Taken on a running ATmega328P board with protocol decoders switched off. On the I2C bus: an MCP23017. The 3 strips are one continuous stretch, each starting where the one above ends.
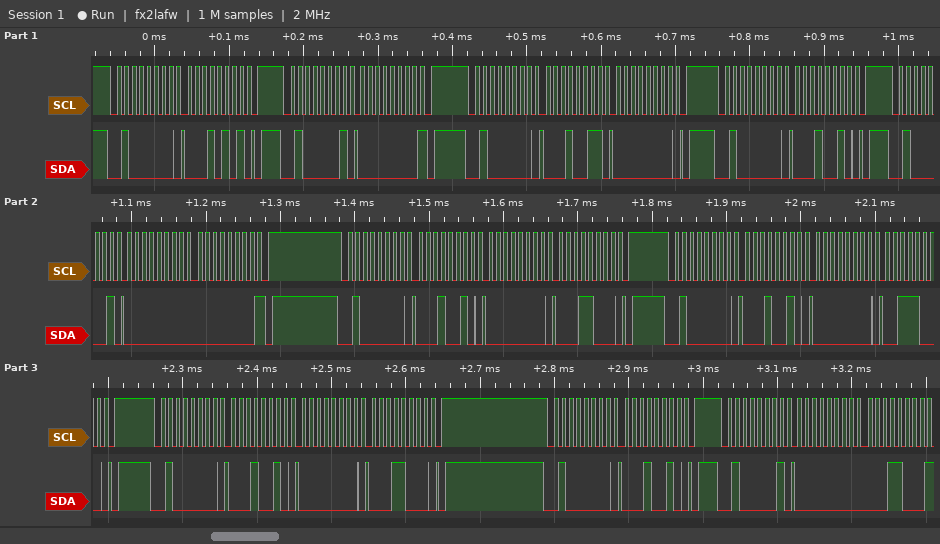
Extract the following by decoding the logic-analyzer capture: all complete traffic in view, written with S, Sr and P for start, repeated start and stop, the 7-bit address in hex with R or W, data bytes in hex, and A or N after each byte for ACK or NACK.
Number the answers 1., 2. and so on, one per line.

1. S 20W A 15 A P S 20R A 00 N P S 20W A 13 A 00 A P S 20W A 12 A P S 20R A 00 A 00 N P S 20W A 12 A 00 A 18 A P S 20W A 12 A 00 A 38 A P S 20W A 12 A 00 A 18 A P S 20W A 12 A P S 20R A 00 A 18 N
